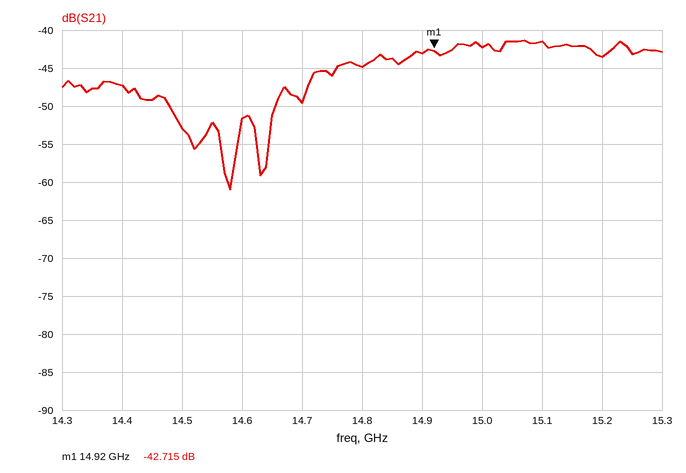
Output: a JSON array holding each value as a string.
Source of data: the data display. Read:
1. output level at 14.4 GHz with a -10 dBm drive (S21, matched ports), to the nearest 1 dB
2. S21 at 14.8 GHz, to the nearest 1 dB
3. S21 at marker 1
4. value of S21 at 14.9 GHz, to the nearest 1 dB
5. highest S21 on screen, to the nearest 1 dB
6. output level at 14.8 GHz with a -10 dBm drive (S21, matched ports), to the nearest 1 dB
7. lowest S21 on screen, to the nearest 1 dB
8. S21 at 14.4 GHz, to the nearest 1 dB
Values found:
["-57 dBm", "-45 dB", "-42.715 dB", "-43 dB", "-41 dB", "-55 dBm", "-61 dB", "-47 dB"]
